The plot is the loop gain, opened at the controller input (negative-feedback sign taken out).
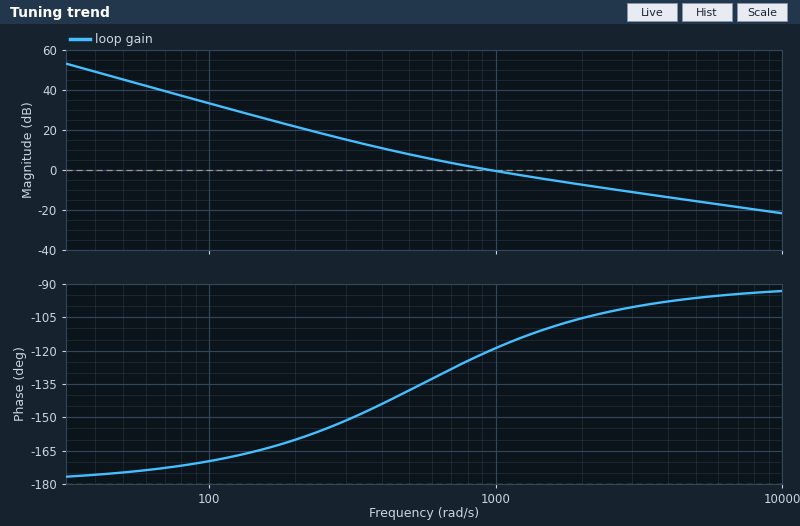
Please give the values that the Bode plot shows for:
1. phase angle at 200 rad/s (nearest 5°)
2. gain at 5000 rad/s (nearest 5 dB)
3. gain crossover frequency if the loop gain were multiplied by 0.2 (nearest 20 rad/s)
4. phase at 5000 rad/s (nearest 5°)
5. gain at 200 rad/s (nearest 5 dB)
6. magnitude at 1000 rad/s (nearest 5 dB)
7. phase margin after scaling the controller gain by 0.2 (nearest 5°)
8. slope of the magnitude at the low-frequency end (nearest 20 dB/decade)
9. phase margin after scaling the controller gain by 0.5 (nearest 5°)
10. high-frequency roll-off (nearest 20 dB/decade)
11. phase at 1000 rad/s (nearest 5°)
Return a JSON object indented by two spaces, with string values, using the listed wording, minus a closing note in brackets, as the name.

{
  "phase angle at 200 rad/s": "-160°",
  "gain at 5000 rad/s": "-15 dB",
  "gain crossover frequency if the loop gain were multiplied by 0.2": "320 rad/s",
  "phase at 5000 rad/s": "-95°",
  "gain at 200 rad/s": "20 dB",
  "magnitude at 1000 rad/s": "0 dB",
  "phase margin after scaling the controller gain by 0.2": "30°",
  "slope of the magnitude at the low-frequency end": "-40 dB/decade",
  "phase margin after scaling the controller gain by 0.5": "45°",
  "high-frequency roll-off": "-20 dB/decade",
  "phase at 1000 rad/s": "-120°"
}
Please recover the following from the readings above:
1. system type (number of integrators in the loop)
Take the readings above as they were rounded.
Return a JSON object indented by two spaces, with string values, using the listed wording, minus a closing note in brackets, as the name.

{
  "system type": "2"
}
